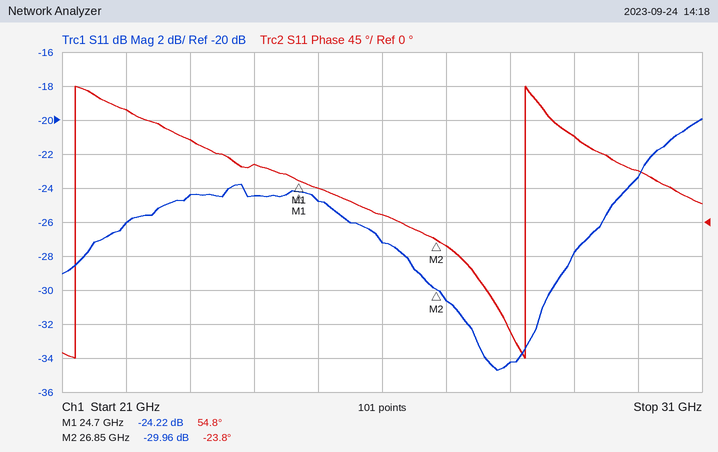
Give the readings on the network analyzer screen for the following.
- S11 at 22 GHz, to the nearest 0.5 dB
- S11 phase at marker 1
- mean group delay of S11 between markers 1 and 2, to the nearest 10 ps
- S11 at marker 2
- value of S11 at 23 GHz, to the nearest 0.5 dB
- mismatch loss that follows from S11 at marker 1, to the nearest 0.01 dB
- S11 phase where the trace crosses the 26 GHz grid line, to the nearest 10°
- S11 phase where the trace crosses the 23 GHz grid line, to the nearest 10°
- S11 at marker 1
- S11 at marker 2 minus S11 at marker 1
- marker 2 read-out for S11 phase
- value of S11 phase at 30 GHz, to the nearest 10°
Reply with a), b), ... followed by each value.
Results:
a) -26.0 dB
b) 54.8°
c) 100 ps
d) -29.96 dB
e) -24.5 dB
f) 0.02 dB
g) 10°
h) 110°
i) -24.22 dB
j) -5.74 dB
k) -23.8°
l) 70°
